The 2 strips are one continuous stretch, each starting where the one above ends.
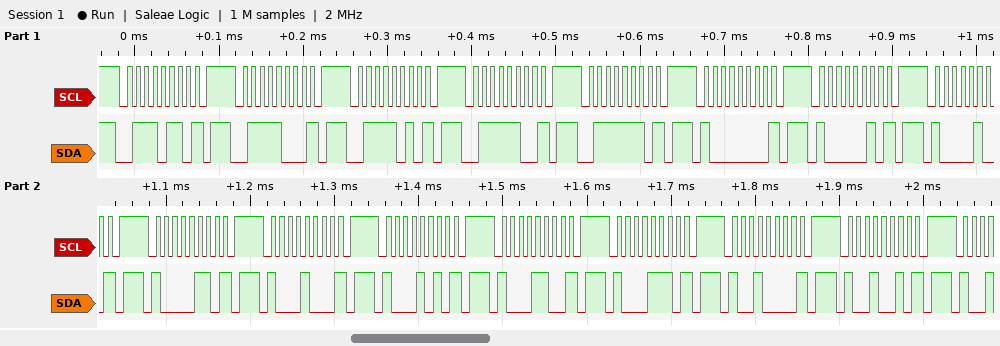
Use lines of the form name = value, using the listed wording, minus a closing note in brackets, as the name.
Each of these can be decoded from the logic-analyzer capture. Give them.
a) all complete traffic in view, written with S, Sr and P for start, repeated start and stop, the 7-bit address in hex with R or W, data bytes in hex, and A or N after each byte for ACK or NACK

all complete traffic in view, written with S, Sr and P for start, repeated start and stop, the 7-bit address in hex with R or W, data bytes in hex, and A or N after each byte for ACK or NACK = S 3BW N P S 3CW N P S 3DW N P S 3EW N P S 3FW N P S 40W N P S 41W N P S 42W N P S 43W N P S 44W N P S 45W N P S 46W N P S 47W N P S 48W N P S 49W N P
